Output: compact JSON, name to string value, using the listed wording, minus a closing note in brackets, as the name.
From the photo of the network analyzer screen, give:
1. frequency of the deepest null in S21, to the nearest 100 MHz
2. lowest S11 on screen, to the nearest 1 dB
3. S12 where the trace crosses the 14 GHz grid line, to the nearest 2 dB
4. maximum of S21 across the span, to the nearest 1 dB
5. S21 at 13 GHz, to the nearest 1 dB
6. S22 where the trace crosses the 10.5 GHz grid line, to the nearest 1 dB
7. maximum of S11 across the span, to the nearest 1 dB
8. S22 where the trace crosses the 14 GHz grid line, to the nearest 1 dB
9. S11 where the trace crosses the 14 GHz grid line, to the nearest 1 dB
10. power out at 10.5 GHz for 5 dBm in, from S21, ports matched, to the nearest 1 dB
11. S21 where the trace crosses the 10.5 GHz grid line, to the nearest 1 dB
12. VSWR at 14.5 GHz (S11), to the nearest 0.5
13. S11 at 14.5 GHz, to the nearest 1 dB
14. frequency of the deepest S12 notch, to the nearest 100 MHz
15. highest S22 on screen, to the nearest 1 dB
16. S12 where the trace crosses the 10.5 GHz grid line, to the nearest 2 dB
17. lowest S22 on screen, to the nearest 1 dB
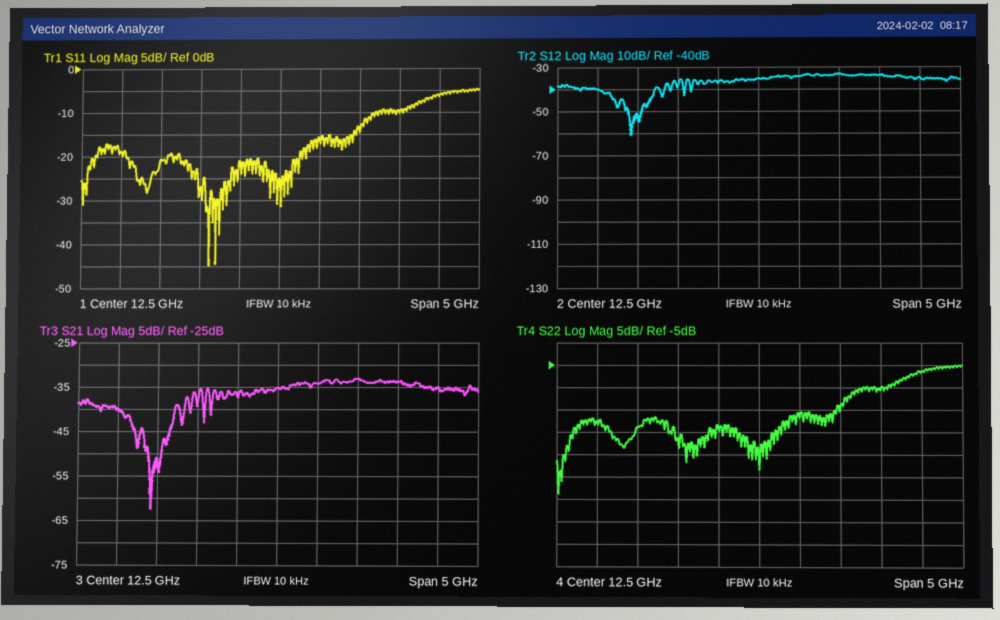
{"frequency of the deepest null in S21, to the nearest 100 MHz": "10.9 GHz", "lowest S11 on screen, to the nearest 1 dB": "-45 dB", "S12 where the trace crosses the 14 GHz grid line, to the nearest 2 dB": "-34 dB", "maximum of S21 across the span, to the nearest 1 dB": "-33 dB", "S21 at 13 GHz, to the nearest 1 dB": "-34 dB", "S22 where the trace crosses the 10.5 GHz grid line, to the nearest 1 dB": "-18 dB", "maximum of S11 across the span, to the nearest 1 dB": "-5 dB", "S22 where the trace crosses the 14 GHz grid line, to the nearest 1 dB": "-10 dB", "S11 where the trace crosses the 14 GHz grid line, to the nearest 1 dB": "-10 dB", "power out at 10.5 GHz for 5 dBm in, from S21, ports matched, to the nearest 1 dB": "-35 dBm", "S21 where the trace crosses the 10.5 GHz grid line, to the nearest 1 dB": "-40 dB", "VSWR at 14.5 GHz (S11), to the nearest 0.5": "3.0", "S11 at 14.5 GHz, to the nearest 1 dB": "-6 dB", "frequency of the deepest S12 notch, to the nearest 100 MHz": "10.9 GHz", "highest S22 on screen, to the nearest 1 dB": "-5 dB", "S12 where the trace crosses the 10.5 GHz grid line, to the nearest 2 dB": "-40 dB", "lowest S22 on screen, to the nearest 1 dB": "-34 dB"}
